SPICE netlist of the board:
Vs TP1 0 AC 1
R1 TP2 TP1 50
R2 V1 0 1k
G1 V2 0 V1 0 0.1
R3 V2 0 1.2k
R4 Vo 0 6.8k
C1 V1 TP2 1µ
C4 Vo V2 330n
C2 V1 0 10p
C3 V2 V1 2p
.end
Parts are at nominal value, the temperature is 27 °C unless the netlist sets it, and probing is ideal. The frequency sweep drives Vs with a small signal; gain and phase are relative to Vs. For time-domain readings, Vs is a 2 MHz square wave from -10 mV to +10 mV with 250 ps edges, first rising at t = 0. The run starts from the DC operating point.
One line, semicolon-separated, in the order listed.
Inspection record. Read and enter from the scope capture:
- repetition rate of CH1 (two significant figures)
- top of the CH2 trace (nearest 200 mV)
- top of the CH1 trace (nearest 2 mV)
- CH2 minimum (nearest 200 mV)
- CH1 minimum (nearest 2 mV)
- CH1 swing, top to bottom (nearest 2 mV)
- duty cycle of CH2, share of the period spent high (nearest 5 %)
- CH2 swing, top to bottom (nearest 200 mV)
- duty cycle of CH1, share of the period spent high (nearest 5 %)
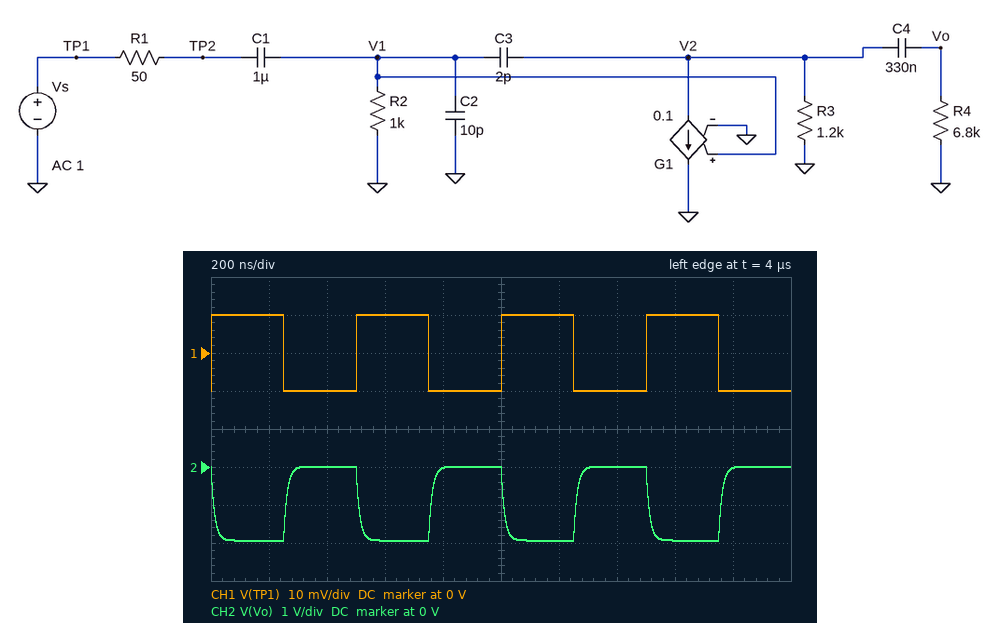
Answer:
2.0 MHz; 0 V; 10 mV; -2.0 V; -10 mV; 20 mV; 50 %; 2.0 V; 50 %
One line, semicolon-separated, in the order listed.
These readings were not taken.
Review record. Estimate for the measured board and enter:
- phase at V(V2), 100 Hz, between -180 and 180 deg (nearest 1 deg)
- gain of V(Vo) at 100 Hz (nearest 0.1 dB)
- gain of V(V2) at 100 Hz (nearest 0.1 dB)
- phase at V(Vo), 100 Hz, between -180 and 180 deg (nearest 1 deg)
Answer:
-128 deg; 33.2 dB; 35.0 dB; -92 deg
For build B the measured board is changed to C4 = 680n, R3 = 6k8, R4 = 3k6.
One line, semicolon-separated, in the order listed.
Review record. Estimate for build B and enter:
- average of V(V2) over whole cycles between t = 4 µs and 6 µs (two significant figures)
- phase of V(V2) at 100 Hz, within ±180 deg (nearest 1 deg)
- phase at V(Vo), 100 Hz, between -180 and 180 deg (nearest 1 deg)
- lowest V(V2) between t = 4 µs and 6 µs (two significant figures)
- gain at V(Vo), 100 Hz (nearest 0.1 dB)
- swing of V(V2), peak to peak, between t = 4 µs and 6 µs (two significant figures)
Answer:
-2.2 V; -144 deg; -111 deg; -4.5 V; 41.6 dB; 4.5 V
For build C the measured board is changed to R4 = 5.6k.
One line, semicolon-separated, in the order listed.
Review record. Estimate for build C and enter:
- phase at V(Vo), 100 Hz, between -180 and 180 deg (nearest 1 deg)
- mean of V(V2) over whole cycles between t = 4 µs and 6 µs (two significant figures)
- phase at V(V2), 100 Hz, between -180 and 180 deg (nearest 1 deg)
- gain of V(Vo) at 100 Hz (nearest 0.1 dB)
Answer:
-88 deg; -940 mV; -129 deg; 32.5 dB
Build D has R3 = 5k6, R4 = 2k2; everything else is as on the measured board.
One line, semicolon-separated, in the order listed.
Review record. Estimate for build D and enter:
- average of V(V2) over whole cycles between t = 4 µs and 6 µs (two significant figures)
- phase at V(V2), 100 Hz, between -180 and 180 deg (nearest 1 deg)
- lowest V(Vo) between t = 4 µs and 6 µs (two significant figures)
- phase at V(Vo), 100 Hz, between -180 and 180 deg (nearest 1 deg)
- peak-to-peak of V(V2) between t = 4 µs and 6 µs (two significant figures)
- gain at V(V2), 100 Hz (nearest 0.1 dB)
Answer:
-1.5 V; -157 deg; -3.0 V; -92 deg; 3.0 V; 44.6 dB
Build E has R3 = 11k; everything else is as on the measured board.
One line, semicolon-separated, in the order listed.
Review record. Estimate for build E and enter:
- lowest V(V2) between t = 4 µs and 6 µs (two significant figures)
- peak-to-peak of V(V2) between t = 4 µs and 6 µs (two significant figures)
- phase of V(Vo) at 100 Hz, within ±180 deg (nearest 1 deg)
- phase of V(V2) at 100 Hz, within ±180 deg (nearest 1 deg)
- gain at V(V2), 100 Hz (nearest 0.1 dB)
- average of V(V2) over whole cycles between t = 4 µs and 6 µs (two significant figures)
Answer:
-7.9 V; 7.9 V; -108 deg; -144 deg; 48.3 dB; -4.0 V
